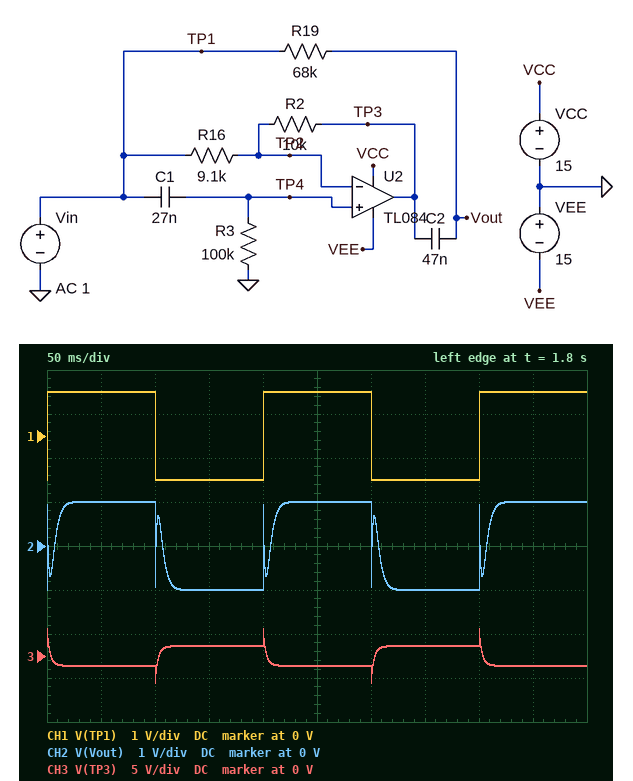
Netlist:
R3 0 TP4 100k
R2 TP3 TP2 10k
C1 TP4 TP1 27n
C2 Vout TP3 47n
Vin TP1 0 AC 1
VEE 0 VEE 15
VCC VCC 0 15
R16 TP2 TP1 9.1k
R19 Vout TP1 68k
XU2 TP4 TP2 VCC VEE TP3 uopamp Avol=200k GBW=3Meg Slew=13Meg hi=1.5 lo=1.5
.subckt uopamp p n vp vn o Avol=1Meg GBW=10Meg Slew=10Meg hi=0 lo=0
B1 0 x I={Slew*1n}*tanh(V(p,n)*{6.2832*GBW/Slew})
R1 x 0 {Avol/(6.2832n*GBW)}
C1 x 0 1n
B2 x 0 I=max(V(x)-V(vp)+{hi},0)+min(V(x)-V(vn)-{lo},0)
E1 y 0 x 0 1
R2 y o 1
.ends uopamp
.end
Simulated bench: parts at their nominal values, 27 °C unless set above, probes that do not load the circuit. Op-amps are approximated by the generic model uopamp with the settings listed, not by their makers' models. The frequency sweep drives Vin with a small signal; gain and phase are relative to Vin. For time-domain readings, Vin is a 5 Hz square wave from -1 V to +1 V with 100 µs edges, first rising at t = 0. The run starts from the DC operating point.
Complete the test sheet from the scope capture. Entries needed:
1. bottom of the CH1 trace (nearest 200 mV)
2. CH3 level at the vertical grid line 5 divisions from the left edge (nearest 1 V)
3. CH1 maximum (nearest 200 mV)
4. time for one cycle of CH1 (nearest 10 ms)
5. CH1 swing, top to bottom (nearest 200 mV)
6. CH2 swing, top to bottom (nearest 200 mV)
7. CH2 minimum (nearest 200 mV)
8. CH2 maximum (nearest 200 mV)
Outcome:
-1.0 V
-1 V
1.0 V
200 ms
2.0 V
2.0 V
-1.0 V
1.0 V
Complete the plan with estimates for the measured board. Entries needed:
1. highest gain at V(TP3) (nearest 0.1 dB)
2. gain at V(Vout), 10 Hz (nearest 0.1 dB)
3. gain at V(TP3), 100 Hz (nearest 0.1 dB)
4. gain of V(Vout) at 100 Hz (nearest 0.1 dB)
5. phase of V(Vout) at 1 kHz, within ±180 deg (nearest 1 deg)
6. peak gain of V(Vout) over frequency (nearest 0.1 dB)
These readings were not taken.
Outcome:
0.8 dB
-0.6 dB
0.2 dB
-5.1 dB
7 deg
0 dB
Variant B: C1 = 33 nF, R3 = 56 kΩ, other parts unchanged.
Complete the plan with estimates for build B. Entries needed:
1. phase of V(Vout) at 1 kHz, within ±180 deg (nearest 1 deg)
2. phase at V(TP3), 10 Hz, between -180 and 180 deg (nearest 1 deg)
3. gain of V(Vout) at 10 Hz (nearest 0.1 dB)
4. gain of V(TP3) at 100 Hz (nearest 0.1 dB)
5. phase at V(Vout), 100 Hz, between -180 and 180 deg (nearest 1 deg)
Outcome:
10 deg
167 deg
-0.4 dB
0.4 dB
105 deg
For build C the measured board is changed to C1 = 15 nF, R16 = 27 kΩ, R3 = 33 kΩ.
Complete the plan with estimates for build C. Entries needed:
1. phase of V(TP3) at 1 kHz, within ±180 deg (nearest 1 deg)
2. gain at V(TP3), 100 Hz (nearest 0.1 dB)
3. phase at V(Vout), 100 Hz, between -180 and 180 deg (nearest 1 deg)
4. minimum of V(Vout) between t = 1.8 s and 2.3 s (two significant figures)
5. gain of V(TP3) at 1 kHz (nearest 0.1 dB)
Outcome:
25 deg
-6.7 dB
-130 deg
-1.0 V
-0.4 dB
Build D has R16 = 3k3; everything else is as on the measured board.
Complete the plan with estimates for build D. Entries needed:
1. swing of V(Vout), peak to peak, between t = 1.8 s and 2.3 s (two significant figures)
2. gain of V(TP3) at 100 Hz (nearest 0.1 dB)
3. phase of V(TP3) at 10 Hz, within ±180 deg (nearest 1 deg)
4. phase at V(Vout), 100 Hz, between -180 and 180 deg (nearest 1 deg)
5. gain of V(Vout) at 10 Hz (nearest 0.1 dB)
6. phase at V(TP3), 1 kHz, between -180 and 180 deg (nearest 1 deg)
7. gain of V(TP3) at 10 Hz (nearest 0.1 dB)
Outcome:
4.5 V
4.9 dB
167 deg
118 deg
0.2 dB
13 deg
9.5 dB
